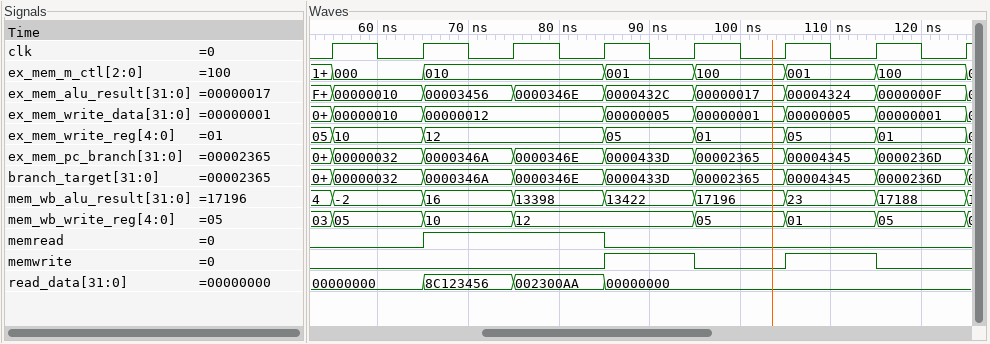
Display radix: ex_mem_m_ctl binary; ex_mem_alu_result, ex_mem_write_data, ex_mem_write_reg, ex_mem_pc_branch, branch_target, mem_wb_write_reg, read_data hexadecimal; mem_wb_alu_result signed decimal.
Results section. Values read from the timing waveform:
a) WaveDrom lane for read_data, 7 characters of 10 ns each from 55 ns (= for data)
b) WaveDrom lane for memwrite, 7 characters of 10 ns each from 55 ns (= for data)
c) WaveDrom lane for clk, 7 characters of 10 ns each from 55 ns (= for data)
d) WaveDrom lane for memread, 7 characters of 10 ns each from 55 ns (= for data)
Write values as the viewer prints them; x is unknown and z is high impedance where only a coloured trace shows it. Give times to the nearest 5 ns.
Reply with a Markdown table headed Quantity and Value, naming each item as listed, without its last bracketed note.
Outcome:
| Quantity | Value |
|---|---|
| WaveDrom lane for read_data, 7 characters of 10 ns each from 55 ns | {name: 'read_data', wave: '====...', data: '00000000 8C123456 002300AA 00000000'} |
| WaveDrom lane for memwrite, 7 characters of 10 ns each from 55 ns | {name: 'memwrite', wave: '0..1010'} |
| WaveDrom lane for clk, 7 characters of 10 ns each from 55 ns | {name: 'clk', wave: 'p......'} |
| WaveDrom lane for memread, 7 characters of 10 ns each from 55 ns | {name: 'memread', wave: '01.0...'} |
